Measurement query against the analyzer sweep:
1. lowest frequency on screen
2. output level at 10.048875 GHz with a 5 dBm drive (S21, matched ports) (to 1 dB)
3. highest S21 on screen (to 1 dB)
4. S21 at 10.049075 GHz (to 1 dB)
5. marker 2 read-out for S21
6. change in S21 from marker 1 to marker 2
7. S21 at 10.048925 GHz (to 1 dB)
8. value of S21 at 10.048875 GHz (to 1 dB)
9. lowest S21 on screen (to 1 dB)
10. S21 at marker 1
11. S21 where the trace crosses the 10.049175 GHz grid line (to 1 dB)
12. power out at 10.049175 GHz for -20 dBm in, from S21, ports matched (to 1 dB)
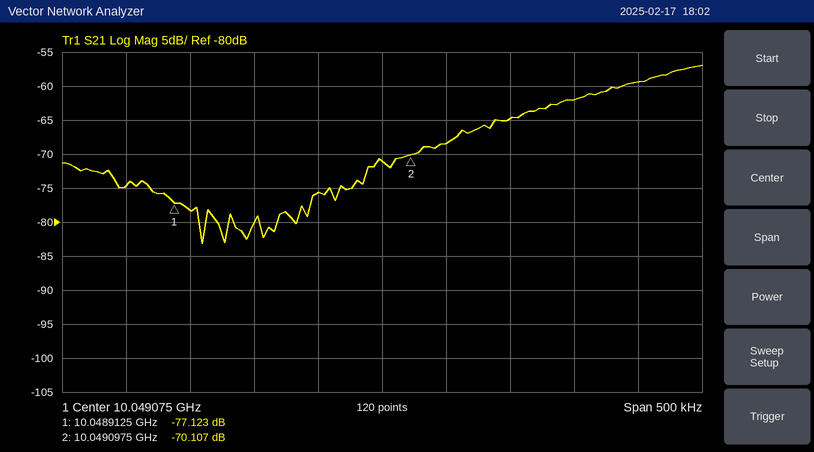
10.048825 GHz
-70 dBm
-57 dB
-71 dB
-70.107 dB
7.016 dB
-78 dB
-75 dB
-83 dB
-77.123 dB
-65 dB
-85 dBm
